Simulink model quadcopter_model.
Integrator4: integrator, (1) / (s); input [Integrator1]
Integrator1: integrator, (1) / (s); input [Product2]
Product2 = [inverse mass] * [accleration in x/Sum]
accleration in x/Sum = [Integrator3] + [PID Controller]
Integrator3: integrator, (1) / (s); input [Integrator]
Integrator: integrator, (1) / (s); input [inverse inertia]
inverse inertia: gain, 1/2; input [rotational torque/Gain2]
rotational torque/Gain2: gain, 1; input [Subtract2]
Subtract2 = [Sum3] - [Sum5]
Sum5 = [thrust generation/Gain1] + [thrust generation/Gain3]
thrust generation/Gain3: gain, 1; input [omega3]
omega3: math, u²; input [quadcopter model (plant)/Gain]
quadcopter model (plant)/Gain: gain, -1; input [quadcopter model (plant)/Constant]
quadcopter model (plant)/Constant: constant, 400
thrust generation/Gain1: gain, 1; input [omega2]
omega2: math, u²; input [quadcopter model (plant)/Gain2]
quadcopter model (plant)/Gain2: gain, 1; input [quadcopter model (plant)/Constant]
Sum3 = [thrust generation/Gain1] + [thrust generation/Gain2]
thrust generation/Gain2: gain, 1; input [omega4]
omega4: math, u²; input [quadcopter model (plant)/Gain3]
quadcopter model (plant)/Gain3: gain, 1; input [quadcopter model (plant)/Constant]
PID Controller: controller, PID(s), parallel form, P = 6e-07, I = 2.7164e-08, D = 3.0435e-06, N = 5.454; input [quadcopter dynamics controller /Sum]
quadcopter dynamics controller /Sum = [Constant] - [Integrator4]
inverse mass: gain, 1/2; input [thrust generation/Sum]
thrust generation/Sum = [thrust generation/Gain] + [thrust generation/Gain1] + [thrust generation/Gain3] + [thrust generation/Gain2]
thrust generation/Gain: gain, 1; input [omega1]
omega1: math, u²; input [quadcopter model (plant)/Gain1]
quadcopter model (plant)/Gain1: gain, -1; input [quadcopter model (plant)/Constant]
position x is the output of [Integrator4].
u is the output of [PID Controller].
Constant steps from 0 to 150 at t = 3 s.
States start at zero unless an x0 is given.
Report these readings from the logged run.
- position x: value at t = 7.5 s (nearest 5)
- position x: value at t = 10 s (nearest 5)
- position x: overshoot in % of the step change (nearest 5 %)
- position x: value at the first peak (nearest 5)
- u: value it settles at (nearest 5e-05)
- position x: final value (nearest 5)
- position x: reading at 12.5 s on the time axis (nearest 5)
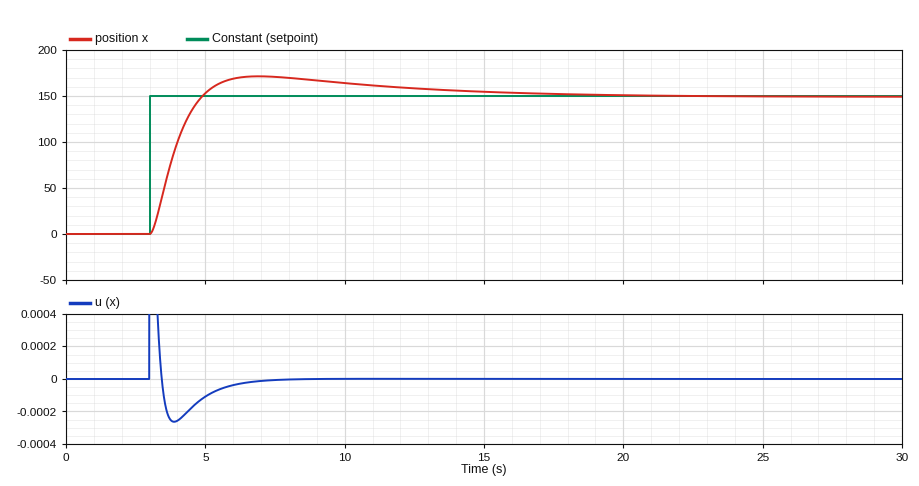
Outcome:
170
165
15 %
170
0.00000
150
160
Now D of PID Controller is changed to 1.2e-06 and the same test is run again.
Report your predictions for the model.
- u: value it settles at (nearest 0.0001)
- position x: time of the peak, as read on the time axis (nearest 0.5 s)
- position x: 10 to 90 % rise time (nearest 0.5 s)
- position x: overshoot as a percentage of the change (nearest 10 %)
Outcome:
0.0000
8.5 s
2.0 s
40 %
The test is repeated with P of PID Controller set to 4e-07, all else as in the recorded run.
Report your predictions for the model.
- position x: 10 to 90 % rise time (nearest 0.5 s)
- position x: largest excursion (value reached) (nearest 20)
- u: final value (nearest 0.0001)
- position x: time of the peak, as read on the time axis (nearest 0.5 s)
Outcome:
1.5 s
160
0.0000
7.5 s
